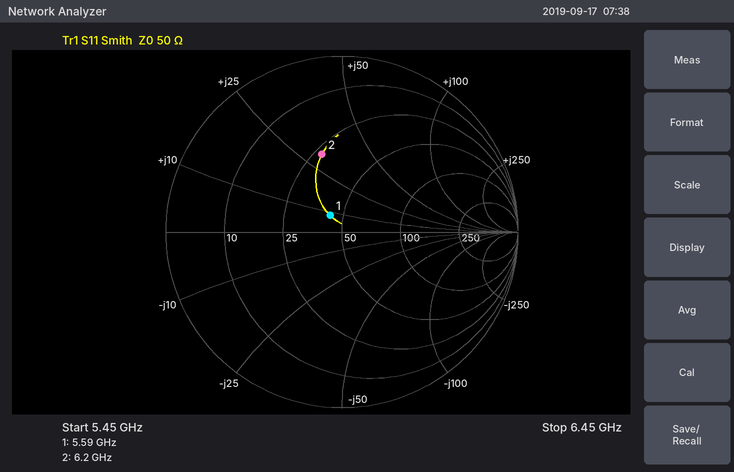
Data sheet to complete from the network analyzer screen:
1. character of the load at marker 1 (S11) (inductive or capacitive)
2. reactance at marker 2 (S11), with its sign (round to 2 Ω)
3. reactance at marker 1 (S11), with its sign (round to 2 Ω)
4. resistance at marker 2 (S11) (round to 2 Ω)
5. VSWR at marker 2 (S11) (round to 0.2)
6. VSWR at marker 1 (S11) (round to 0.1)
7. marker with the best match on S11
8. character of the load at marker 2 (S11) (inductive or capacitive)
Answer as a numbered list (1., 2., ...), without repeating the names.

1. inductive
2. +30 Ω
3. +8 Ω
4. 28 Ω
5. 2.6
6. 1.3
7. marker 1
8. inductive
